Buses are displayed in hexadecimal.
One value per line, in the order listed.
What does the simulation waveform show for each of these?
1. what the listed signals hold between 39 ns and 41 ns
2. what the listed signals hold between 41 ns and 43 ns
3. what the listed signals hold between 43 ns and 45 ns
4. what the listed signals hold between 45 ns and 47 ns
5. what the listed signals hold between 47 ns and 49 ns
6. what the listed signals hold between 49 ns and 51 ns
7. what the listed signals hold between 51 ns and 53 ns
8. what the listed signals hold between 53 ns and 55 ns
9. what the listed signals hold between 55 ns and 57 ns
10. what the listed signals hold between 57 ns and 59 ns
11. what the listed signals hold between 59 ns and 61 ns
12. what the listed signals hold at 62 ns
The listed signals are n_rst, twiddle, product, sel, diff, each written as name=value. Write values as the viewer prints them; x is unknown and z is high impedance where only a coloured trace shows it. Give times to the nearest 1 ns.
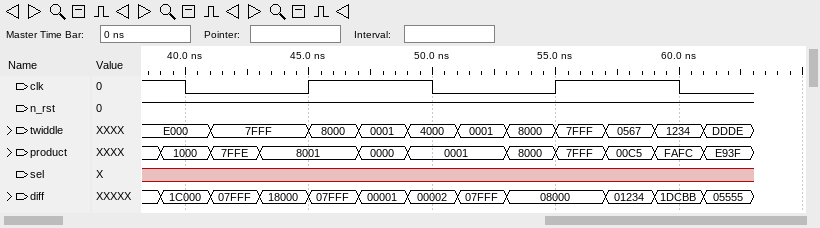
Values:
n_rst=1, twiddle=E000, product=1000, sel=x, diff=1C000
n_rst=1, twiddle=7FFF, product=7FFE, sel=x, diff=07FFF
n_rst=1, twiddle=7FFF, product=8001, sel=x, diff=18000
n_rst=1, twiddle=8000, product=8001, sel=x, diff=07FFF
n_rst=1, twiddle=0001, product=0000, sel=x, diff=00001
n_rst=1, twiddle=4000, product=0001, sel=x, diff=00002
n_rst=1, twiddle=0001, product=0001, sel=x, diff=07FFF
n_rst=1, twiddle=8000, product=8000, sel=x, diff=08000
n_rst=1, twiddle=7FFF, product=7FFF, sel=x, diff=08000
n_rst=1, twiddle=0567, product=00C5, sel=x, diff=01234
n_rst=1, twiddle=1234, product=FAFC, sel=x, diff=1DCBB
n_rst=1, twiddle=DDDE, product=E93F, sel=x, diff=05555
